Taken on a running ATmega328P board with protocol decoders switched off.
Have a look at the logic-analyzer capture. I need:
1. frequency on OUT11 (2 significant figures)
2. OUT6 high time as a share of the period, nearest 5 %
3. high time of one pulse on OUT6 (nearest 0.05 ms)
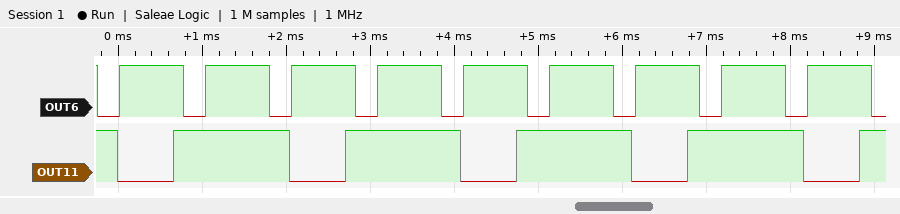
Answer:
490 Hz
75 %
0.75 ms
